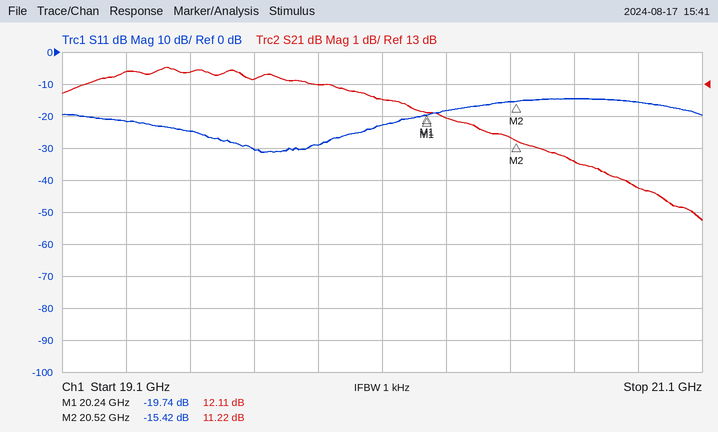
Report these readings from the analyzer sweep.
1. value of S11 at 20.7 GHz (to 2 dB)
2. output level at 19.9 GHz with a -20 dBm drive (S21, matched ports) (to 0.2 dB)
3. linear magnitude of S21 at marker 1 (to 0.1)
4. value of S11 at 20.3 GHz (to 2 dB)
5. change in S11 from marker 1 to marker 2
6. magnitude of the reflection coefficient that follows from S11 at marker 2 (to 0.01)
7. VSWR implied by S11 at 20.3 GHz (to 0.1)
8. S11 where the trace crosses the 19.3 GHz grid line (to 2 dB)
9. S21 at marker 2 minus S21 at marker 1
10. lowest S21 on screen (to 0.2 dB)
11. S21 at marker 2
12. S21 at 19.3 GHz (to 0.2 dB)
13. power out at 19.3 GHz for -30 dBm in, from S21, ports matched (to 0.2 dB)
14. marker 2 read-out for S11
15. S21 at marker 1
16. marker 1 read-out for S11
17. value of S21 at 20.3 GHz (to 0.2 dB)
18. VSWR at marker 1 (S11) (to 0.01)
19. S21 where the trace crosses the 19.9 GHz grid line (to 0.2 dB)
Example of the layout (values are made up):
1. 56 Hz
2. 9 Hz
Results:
1. -14 dB
2. -7.0 dBm
3. 4.0
4. -18 dB
5. 4.32 dB
6. 0.17
7. 1.3
8. -22 dB
9. -0.89 dB
10. 8.8 dB
11. 11.22 dB
12. 13.4 dB
13. -16.6 dBm
14. -15.42 dB
15. 12.11 dB
16. -19.74 dB
17. 12.0 dB
18. 1.23
19. 13.0 dB
